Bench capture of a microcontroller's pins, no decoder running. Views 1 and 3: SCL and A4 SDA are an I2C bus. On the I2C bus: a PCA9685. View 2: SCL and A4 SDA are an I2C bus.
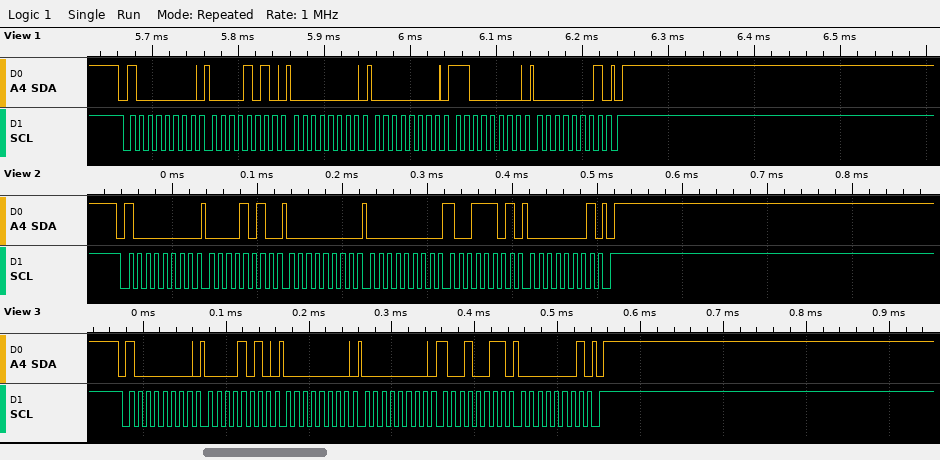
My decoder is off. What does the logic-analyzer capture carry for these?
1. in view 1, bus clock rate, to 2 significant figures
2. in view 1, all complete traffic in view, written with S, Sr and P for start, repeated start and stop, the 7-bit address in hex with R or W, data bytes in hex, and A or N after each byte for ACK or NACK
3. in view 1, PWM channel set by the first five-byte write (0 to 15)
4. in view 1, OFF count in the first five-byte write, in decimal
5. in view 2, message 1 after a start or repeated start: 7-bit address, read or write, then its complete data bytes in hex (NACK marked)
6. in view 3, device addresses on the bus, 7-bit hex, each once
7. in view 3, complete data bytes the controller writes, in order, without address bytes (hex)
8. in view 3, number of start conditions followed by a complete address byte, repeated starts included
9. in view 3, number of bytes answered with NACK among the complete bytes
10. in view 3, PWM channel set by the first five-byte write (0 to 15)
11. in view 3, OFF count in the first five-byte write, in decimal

100 kHz
S 40W A 0A A 00 A 00 A C0 A 01 A P
1
448
0x40 write: 0A 00 00 9D 01
0x40
0A 00 00 93 01
1
0
1
403
